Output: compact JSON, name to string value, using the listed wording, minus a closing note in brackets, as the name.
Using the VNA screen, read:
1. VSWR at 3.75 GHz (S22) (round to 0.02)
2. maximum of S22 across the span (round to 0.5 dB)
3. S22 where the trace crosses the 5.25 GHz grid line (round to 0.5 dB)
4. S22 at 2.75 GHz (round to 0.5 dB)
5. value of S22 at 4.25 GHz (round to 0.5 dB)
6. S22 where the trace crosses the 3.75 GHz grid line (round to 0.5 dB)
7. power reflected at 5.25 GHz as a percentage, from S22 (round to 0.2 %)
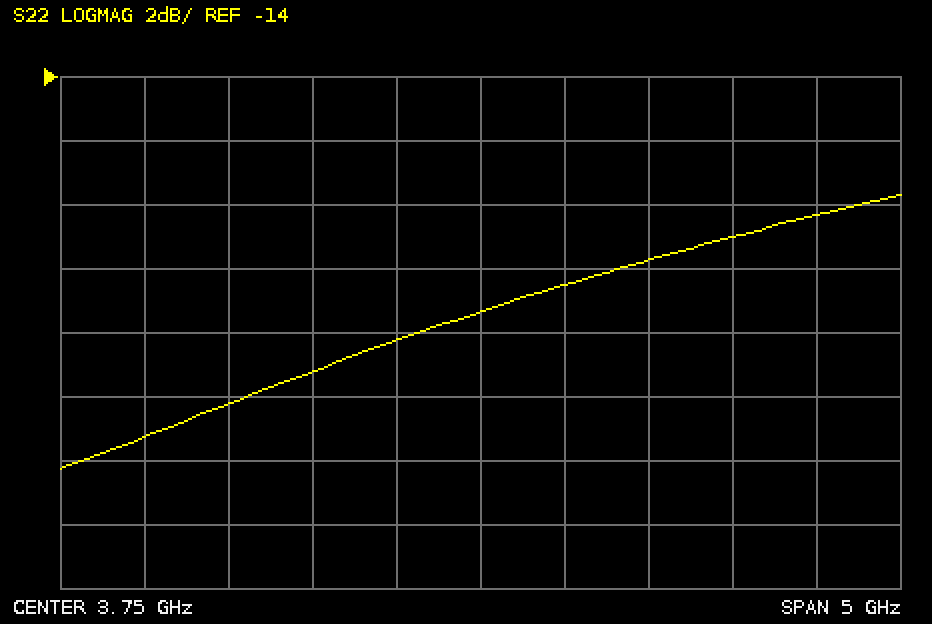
{"VSWR at 3.75 GHz (S22)": "1.18", "maximum of S22 across the span": "-17.5 dB", "S22 where the trace crosses the 5.25 GHz grid line": "-19.0 dB", "S22 at 2.75 GHz": "-23.0 dB", "value of S22 at 4.25 GHz": "-20.5 dB", "S22 where the trace crosses the 3.75 GHz grid line": "-21.5 dB", "power reflected at 5.25 GHz as a percentage, from S22": "1.2 %"}
